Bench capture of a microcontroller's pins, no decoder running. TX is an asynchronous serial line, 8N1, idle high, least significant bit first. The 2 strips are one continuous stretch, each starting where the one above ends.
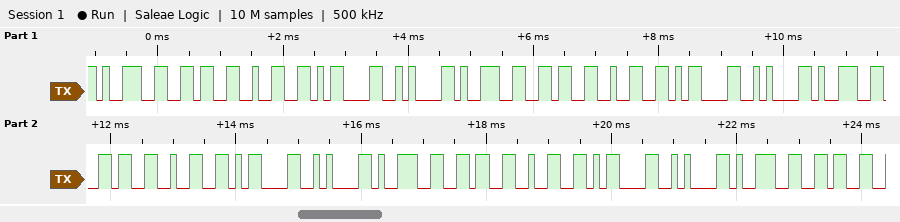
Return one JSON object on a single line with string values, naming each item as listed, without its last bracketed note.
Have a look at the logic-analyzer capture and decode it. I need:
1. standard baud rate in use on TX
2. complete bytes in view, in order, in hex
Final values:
{"standard baud rate in use on TX": "9600 baud", "complete bytes in view, in order, in hex": "0x39 0x36 0x32 0x0D 0x0A 0x39 0x36 0x32 0x0D 0x0A 0x39 0x36 0x32 0x0D 0x0A 0x39 0x36 0x32 0x0D 0x0A 0x39 0x36"}
